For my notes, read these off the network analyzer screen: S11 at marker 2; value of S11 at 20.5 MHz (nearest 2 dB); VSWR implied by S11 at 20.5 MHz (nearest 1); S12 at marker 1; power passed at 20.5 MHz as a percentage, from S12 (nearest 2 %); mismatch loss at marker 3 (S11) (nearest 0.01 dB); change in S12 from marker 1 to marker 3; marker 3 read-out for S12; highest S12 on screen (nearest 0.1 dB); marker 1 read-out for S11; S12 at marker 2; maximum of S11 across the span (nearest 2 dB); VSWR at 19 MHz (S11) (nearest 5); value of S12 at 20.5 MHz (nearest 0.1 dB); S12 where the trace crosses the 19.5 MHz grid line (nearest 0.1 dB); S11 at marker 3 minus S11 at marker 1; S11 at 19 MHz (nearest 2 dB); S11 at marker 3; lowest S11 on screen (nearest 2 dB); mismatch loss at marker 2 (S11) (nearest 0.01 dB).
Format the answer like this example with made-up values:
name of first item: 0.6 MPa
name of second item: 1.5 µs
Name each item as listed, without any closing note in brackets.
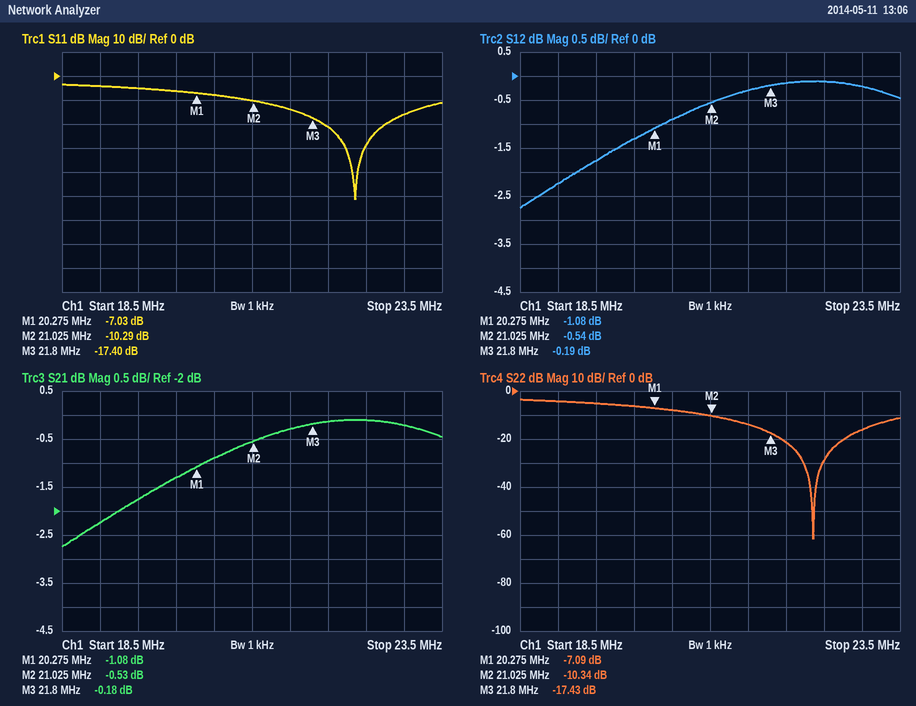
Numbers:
S11 at marker 2: -10.29 dB
value of S11 at 20.5 MHz: -8 dB
VSWR implied by S11 at 20.5 MHz: 2
S12 at marker 1: -1.08 dB
power passed at 20.5 MHz as a percentage, from S12: 82 %
mismatch loss at marker 3 (S11): 0.08 dB
change in S12 from marker 1 to marker 3: 0.89 dB
marker 3 read-out for S12: -0.19 dB
highest S12 on screen: -0.1 dB
marker 1 read-out for S11: -7.03 dB
S12 at marker 2: -0.54 dB
maximum of S11 across the span: -4 dB
VSWR at 19 MHz (S11): 5
value of S12 at 20.5 MHz: -0.9 dB
S12 where the trace crosses the 19.5 MHz grid line: -1.8 dB
S11 at marker 3 minus S11 at marker 1: -10.37 dB
S11 at 19 MHz: -4 dB
S11 at marker 3: -17.40 dB
lowest S11 on screen: -52 dB
mismatch loss at marker 2 (S11): 0.43 dB
